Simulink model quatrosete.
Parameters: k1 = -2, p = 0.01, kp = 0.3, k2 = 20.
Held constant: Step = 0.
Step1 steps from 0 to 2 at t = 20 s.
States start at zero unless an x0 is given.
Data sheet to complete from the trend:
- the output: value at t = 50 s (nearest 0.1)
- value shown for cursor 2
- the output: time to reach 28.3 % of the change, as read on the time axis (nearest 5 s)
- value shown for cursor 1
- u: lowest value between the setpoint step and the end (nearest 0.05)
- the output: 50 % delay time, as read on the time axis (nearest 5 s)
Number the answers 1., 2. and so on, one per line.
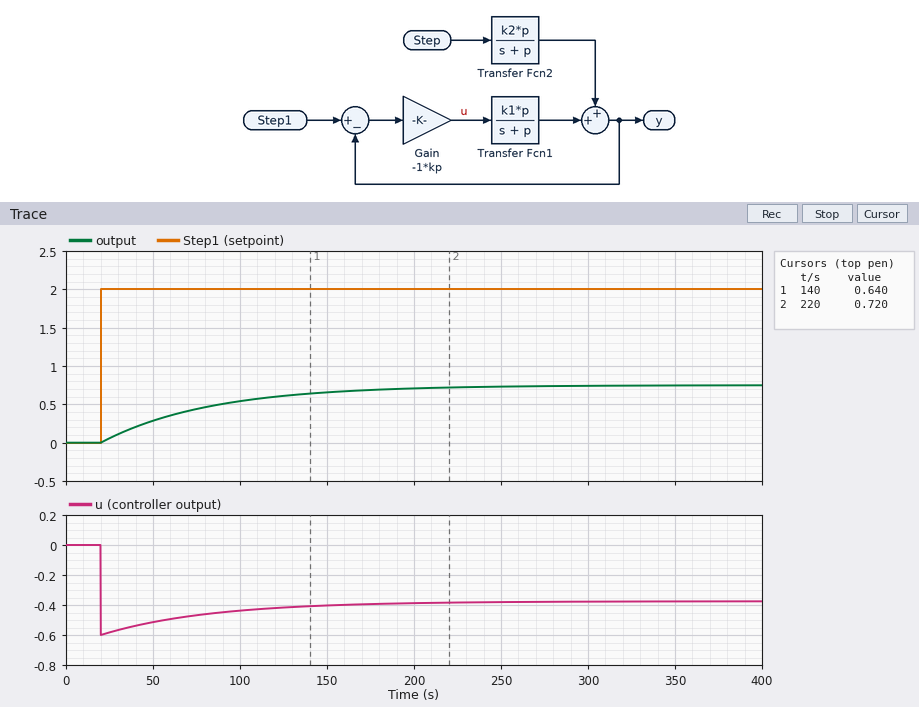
1. 0.3
2. 0.720
3. 40 s
4. 0.640
5. -0.60
6. 65 s
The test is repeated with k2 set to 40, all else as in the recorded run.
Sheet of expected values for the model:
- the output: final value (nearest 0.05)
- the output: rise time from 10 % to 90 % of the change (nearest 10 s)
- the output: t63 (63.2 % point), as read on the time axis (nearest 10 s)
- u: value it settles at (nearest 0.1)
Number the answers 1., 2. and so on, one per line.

1. 0.75
2. 140 s
3. 80 s
4. -0.4
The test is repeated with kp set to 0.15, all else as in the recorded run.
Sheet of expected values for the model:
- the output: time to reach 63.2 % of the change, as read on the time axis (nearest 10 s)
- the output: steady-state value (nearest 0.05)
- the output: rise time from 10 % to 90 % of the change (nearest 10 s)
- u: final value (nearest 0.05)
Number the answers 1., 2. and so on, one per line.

1. 100 s
2. 0.45
3. 170 s
4. -0.25
